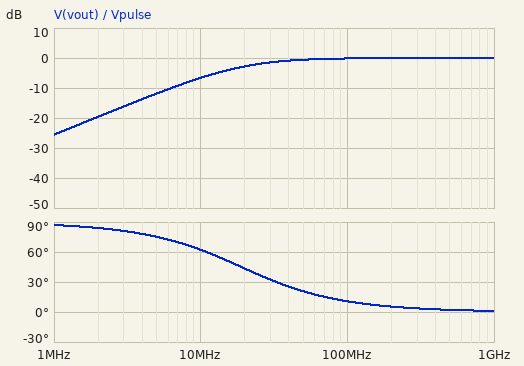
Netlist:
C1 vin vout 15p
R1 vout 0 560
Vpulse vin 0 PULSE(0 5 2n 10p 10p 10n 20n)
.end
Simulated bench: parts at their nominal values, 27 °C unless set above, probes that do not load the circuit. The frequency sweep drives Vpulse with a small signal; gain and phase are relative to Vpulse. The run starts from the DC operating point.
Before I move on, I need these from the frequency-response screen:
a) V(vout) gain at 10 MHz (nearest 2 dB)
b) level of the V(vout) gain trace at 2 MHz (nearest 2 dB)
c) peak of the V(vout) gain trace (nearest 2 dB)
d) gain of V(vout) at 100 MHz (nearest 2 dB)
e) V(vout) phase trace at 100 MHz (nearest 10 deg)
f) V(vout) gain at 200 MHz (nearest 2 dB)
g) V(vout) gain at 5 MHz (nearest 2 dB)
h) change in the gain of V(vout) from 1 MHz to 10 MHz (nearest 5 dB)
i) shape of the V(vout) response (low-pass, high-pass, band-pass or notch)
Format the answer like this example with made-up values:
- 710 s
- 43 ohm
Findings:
- -6 dB
- -20 dB
- 0 dB
- 0 dB
- 10 deg
- 0 dB
- -12 dB
- 20 dB
- high-pass
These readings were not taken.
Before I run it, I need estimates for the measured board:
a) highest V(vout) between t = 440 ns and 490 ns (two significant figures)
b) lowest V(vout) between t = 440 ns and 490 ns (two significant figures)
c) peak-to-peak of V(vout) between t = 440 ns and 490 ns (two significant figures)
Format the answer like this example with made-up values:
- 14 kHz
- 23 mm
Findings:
- 3.8 V
- -3.8 V
- 7.7 V
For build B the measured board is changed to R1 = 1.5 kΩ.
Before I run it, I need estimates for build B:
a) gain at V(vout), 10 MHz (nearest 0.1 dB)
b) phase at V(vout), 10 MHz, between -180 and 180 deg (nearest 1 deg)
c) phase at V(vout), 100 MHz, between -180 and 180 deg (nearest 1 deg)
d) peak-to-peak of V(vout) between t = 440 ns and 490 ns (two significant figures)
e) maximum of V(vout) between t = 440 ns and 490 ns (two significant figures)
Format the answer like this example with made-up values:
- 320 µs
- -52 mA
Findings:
- -1.8 dB
- 35 deg
- 4 deg
- 6.1 V
- 3.0 V
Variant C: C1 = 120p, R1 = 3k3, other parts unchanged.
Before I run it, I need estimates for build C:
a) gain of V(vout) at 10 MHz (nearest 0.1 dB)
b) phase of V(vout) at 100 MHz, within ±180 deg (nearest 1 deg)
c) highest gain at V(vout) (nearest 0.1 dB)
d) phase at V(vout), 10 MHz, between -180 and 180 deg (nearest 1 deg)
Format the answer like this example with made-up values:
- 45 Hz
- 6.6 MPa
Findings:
- 0 dB
- 0 deg
- 0 dB
- 2 deg
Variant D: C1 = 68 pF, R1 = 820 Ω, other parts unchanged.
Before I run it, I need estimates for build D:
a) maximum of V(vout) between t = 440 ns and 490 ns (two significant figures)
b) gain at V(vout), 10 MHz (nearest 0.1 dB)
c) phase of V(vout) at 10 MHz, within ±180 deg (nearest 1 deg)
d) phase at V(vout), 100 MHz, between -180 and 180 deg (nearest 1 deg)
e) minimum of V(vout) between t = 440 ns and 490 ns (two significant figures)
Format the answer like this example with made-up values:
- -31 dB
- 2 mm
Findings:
- 2.7 V
- -0.3 dB
- 16 deg
- 2 deg
- -2.7 V
